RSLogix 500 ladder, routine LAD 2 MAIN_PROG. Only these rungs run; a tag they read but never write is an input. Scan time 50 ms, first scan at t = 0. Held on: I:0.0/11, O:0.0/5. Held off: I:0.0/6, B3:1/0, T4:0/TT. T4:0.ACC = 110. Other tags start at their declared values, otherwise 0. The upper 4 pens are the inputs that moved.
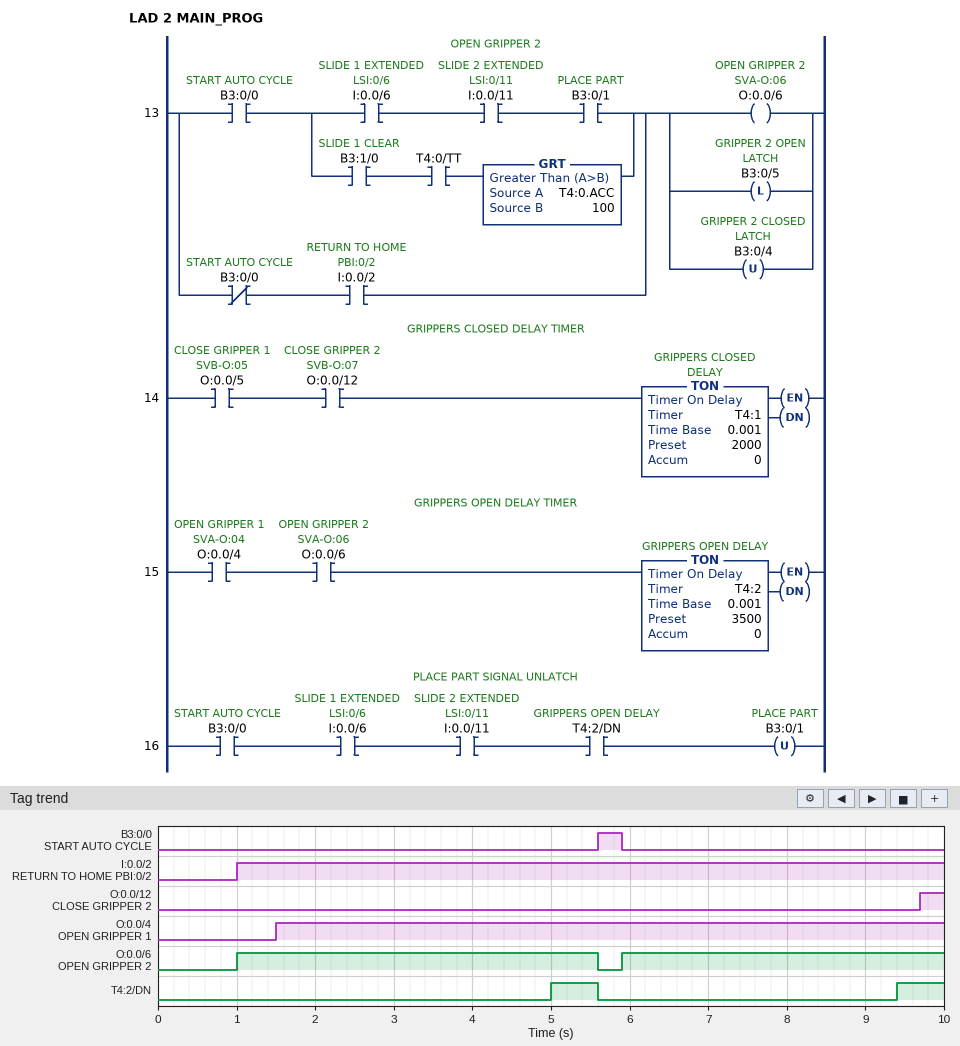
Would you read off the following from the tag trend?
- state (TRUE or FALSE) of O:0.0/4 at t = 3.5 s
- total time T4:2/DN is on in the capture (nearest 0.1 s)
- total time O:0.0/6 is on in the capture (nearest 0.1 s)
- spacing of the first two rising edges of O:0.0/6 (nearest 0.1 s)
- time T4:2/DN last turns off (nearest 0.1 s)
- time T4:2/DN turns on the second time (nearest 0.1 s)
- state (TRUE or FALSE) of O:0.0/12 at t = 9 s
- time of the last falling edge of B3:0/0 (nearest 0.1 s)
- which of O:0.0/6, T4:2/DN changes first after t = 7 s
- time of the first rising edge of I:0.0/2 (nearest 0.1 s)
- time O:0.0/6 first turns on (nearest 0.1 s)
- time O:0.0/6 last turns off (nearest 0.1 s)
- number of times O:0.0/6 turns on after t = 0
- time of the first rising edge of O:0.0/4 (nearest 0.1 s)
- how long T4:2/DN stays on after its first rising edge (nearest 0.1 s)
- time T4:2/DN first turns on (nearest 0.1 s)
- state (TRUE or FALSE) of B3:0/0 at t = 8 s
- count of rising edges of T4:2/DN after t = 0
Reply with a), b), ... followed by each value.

a) TRUE
b) 1.2 s
c) 8.7 s
d) 4.9 s
e) 5.6 s
f) 9.4 s
g) FALSE
h) 5.9 s
i) T4:2/DN
j) 1.0 s
k) 1.0 s
l) 5.6 s
m) 2
n) 1.5 s
o) 0.6 s
p) 5.0 s
q) FALSE
r) 2
